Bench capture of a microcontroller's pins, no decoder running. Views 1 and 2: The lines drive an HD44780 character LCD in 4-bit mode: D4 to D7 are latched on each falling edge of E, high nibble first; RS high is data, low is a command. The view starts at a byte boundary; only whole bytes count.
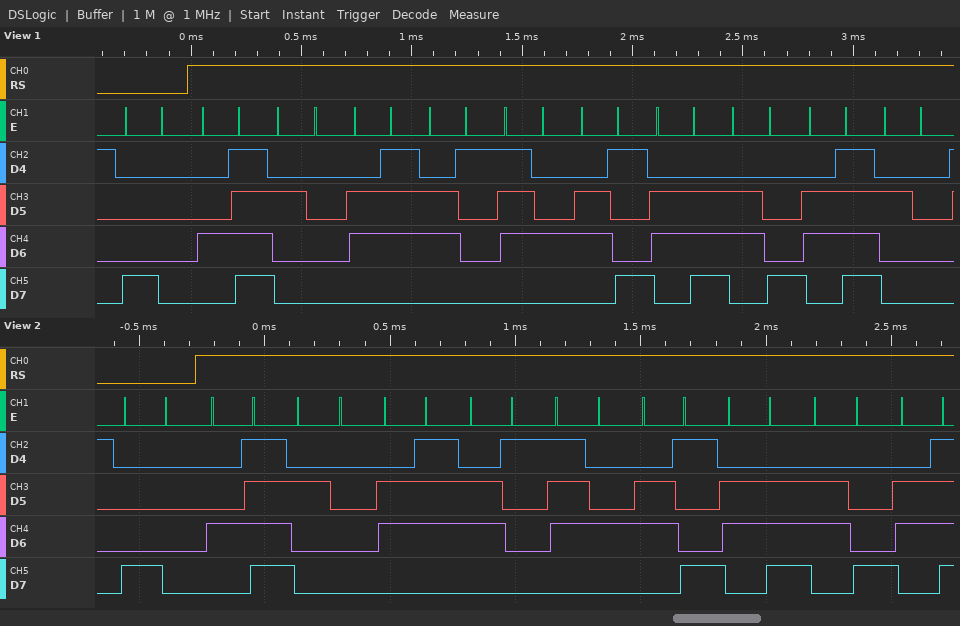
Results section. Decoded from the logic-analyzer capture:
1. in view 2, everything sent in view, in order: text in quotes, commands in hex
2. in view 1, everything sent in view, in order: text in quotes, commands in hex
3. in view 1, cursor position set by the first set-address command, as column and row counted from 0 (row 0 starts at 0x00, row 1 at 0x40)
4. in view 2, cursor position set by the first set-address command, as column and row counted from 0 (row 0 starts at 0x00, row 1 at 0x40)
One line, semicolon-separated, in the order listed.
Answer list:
0x80 "O gatinho"; 0x80 "O gatinho "; column 0, row 0; column 0, row 0
